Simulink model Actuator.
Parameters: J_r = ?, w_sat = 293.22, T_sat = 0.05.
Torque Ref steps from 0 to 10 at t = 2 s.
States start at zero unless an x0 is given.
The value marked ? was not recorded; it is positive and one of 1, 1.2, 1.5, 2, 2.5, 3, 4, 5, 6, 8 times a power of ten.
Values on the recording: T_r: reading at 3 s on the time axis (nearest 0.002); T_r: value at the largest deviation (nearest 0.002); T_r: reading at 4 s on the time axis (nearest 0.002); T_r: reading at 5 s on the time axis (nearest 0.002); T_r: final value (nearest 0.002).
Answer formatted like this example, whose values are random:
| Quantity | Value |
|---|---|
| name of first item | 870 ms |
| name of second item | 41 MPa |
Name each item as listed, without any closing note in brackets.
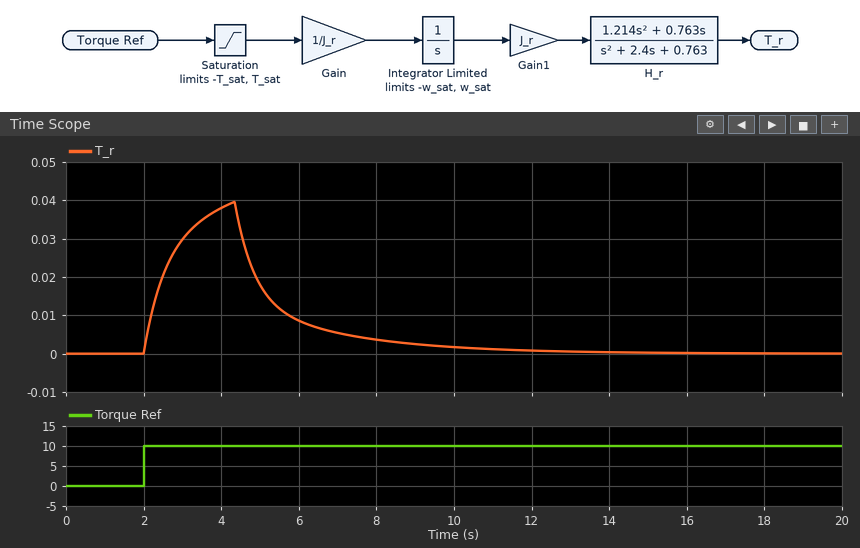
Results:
| Quantity | Value |
|---|---|
| T_r: reading at 3 s on the time axis | 0.030 |
| T_r: value at the largest deviation | 0.040 |
| T_r: reading at 4 s on the time axis | 0.038 |
| T_r: reading at 5 s on the time axis | 0.018 |
| T_r: final value | 0.000 |
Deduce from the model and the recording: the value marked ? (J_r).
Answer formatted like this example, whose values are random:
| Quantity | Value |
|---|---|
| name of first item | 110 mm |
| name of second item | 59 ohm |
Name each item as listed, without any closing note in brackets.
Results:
| Quantity | Value |
|---|---|
| the value marked ? | 0.0004 |
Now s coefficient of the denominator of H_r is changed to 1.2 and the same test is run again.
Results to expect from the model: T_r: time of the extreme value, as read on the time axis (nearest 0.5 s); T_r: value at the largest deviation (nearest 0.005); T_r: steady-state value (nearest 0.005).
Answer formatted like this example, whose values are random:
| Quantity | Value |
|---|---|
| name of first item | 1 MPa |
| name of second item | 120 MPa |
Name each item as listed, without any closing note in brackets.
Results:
| Quantity | Value |
|---|---|
| T_r: time of the extreme value, as read on the time axis | 4.5 s |
| T_r: value at the largest deviation | 0.060 |
| T_r: steady-state value | 0.000 |
